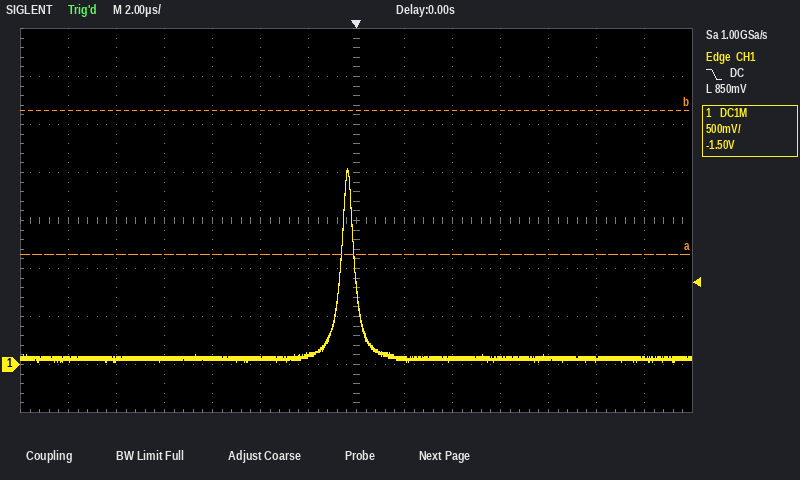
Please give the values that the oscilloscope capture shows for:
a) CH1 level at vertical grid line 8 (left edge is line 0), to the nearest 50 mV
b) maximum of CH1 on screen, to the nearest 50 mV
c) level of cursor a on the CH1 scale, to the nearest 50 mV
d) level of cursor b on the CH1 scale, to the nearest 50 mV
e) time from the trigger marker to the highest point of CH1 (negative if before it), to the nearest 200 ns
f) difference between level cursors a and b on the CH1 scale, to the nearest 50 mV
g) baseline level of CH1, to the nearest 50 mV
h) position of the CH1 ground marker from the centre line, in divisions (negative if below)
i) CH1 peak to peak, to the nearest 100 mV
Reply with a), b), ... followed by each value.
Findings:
a) 50 mV
b) 2.05 V
c) 1.15 V
d) 2.65 V
e) -400 ns
f) 1.50 V
g) 50 mV
h) -3.0 div
i) 2.00 V
